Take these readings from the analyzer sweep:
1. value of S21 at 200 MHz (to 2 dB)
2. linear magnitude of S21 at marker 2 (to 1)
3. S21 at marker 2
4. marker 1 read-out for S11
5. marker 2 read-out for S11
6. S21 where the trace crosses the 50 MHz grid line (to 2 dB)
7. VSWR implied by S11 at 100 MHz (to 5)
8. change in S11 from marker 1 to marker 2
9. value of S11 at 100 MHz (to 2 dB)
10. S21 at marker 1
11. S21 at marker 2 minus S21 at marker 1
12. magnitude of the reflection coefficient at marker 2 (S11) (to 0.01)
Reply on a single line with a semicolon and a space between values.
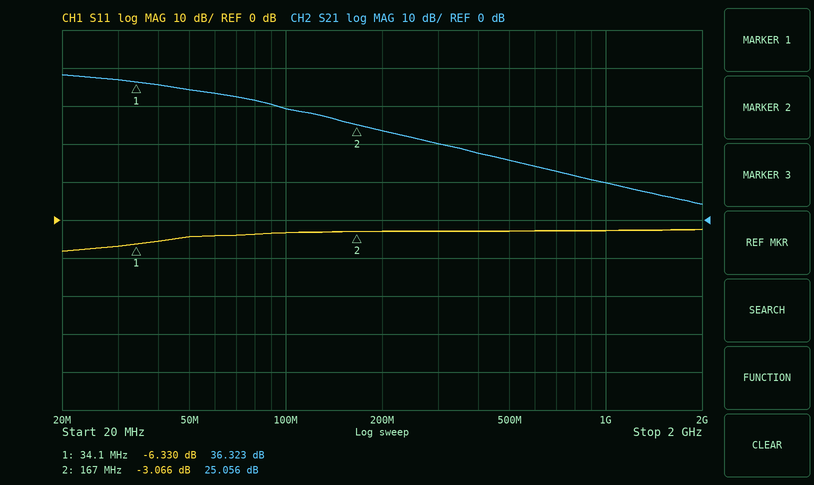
24 dB; 18; 25.056 dB; -6.330 dB; -3.066 dB; 34 dB; 5; 3.264 dB; -4 dB; 36.323 dB; -11.267 dB; 0.70
